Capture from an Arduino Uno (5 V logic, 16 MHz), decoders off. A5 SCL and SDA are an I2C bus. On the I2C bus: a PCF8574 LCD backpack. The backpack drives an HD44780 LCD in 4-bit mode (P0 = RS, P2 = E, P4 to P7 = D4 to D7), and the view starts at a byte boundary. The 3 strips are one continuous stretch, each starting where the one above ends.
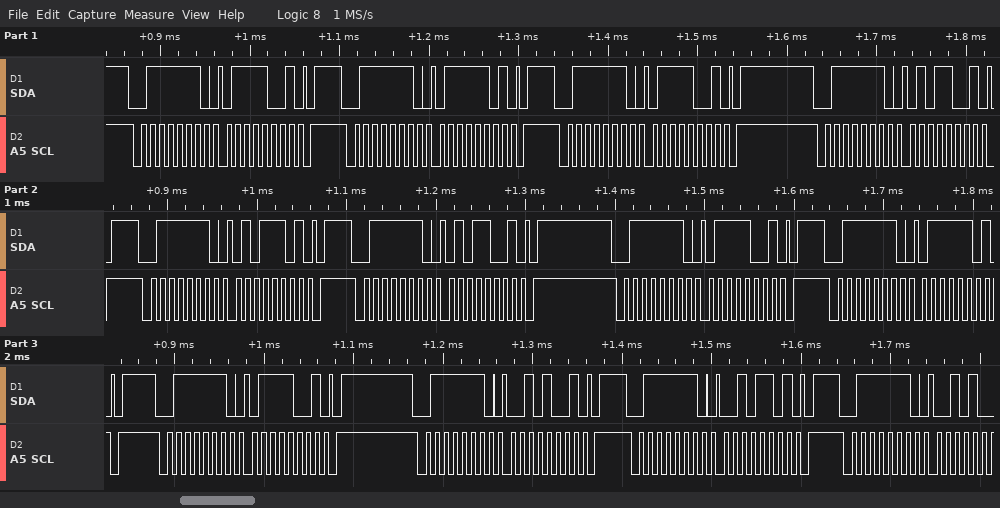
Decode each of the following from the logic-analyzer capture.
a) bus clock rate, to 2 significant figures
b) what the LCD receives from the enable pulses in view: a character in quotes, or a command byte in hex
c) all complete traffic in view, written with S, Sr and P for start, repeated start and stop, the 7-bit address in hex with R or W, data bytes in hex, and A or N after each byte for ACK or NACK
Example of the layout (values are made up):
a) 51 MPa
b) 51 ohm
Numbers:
a) 100 kHz
b) 'u'
c) S 3FW A 79 A P S 3FW A 7D A P S 3FW A 79 A P S 3FW A 59 A P S 3FW A 5D A P S 3FW A 59 A P S 3FW A 79 A P S 3FW A 7D A P S 3FW A 79 A P S 3FW A 29 A P S 3FW A 2D A P S 3FW A
